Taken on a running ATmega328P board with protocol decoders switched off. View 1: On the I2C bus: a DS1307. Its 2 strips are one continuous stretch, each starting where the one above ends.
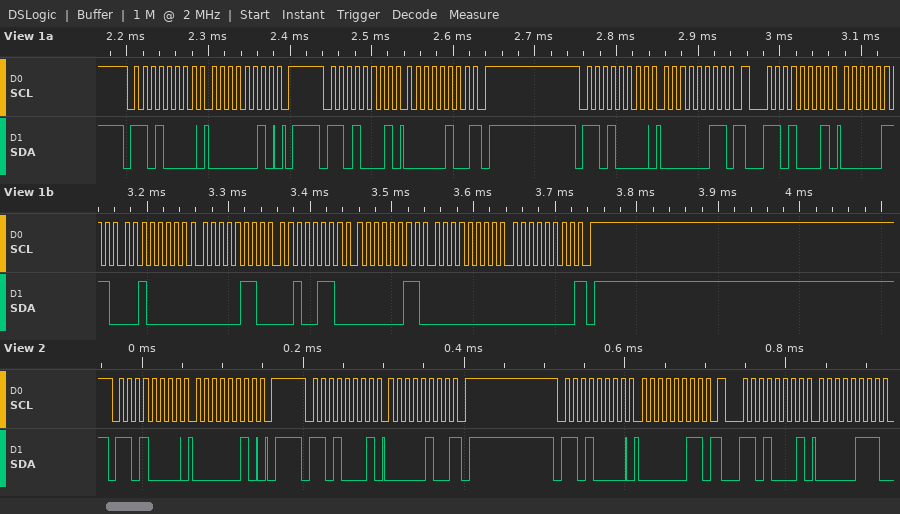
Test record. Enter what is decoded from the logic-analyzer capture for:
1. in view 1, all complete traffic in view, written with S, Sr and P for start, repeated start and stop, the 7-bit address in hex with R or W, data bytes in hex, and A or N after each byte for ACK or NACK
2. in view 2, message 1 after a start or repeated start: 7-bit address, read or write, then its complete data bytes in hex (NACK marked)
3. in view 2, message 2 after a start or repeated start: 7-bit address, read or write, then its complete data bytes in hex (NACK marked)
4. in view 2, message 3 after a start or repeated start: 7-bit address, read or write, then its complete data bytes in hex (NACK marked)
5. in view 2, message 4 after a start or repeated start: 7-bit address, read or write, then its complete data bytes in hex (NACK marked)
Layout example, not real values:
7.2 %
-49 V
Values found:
S 68W A 02 A P S 68R A 04 N P S 68W A 03 A Sr 68R A 07 A 20 A 06 A 26 A 03 A 00 A 00 N P
0x68 write: 02
0x68 read: 04 NACK
0x68 write: 03
0x68 read: 07
